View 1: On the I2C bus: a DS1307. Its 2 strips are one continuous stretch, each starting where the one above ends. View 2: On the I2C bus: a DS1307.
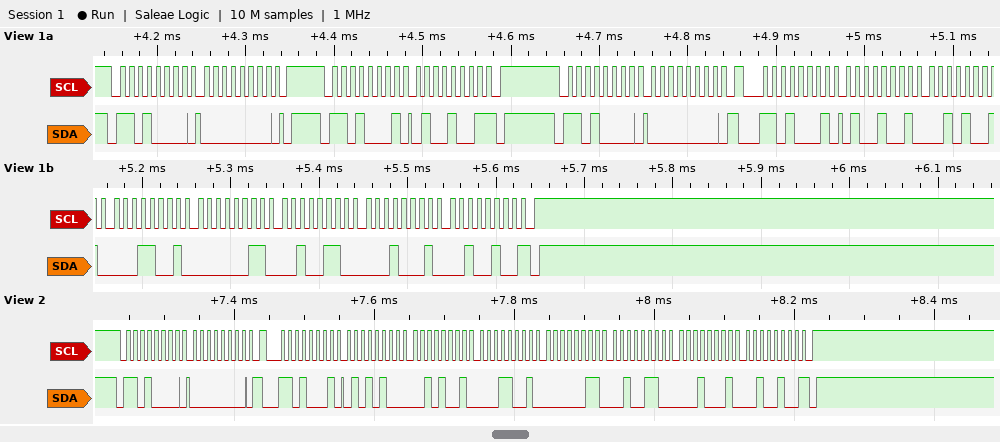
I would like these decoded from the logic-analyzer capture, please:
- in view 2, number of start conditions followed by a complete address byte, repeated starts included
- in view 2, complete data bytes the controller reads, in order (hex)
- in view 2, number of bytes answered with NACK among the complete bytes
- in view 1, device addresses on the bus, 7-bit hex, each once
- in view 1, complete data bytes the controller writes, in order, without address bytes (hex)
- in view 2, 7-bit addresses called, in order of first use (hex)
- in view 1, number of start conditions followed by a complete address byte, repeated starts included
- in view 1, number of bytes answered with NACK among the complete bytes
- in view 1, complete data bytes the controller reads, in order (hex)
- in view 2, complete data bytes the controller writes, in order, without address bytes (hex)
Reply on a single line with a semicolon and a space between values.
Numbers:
2; 54 29 19 03 26 11 24; 1; 0x68; 00 00; 0x68; 4; 2; 49 49 29 19 03 26 11 24; 00
